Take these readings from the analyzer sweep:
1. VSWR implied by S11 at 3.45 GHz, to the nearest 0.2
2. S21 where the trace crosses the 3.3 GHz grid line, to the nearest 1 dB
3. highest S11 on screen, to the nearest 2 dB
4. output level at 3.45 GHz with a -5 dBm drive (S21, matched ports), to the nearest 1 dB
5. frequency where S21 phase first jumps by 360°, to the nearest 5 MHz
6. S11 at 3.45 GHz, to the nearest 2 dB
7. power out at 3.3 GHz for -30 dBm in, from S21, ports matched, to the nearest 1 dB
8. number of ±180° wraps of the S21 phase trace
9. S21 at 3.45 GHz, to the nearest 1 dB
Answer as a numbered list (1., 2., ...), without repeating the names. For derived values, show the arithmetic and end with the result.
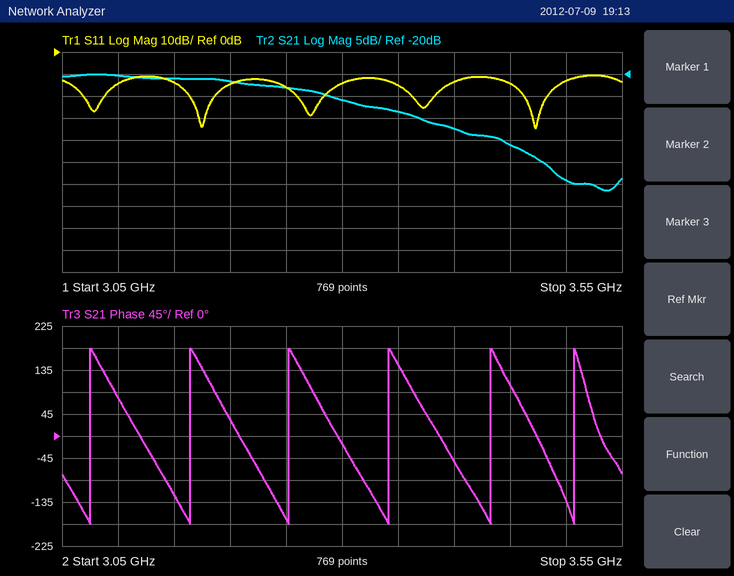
1. |Γ| = 10^(-14/20) = 0.1995; VSWR = (1 + 0.1995)/(1 − 0.1995) ≈ 1.50, so 1.4 to the nearest 0.2
2. -26 dB
3. -10 dB
4. -5 dBm + (-36 dB) = -41 dBm
5. 3.075 GHz
6. -14 dB
7. -30 dBm + (-26 dB) = -56 dBm
8. 6
9. -36 dB
